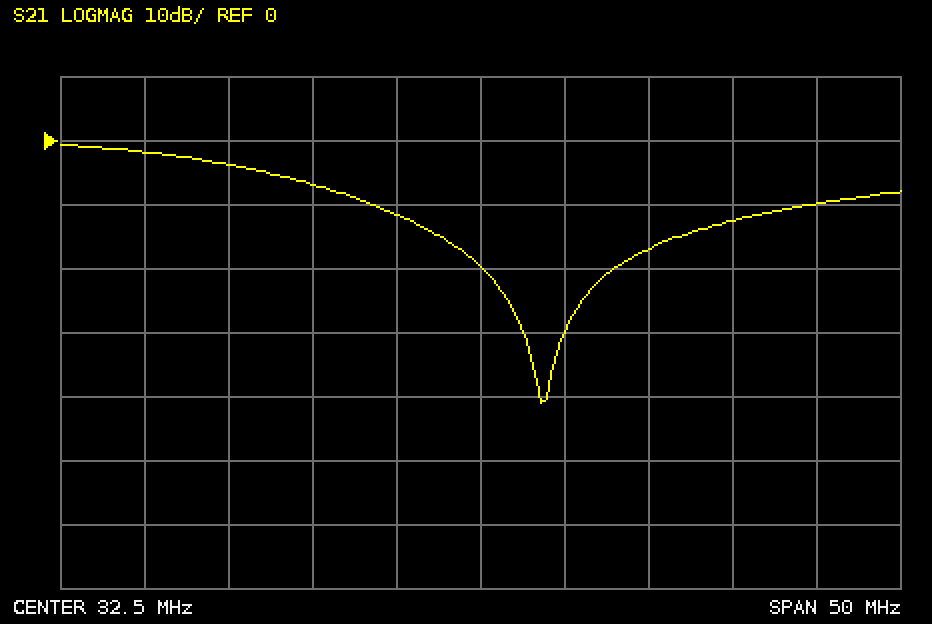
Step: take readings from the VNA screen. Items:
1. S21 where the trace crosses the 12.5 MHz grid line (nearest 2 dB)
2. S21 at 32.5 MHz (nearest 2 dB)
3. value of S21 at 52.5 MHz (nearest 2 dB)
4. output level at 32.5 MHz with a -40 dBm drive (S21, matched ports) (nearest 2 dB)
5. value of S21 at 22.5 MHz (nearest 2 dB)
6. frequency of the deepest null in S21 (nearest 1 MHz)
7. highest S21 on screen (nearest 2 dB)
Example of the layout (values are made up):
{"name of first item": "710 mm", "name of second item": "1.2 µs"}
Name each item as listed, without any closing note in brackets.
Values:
{"S21 where the trace crosses the 12.5 MHz grid line": "-2 dB", "S21 at 32.5 MHz": "-20 dB", "value of S21 at 52.5 MHz": "-10 dB", "output level at 32.5 MHz with a -40 dBm drive (S21, matched ports)": "-60 dBm", "value of S21 at 22.5 MHz": "-6 dB", "frequency of the deepest null in S21": "36 MHz", "highest S21 on screen": "0 dB"}
